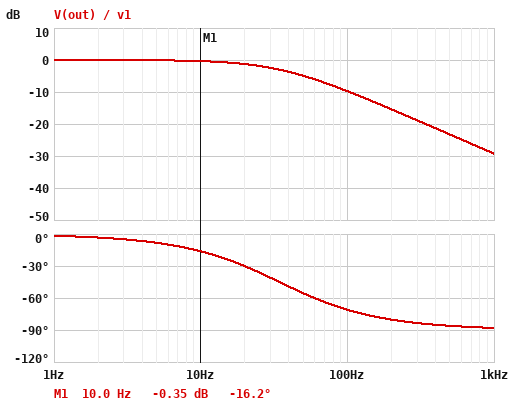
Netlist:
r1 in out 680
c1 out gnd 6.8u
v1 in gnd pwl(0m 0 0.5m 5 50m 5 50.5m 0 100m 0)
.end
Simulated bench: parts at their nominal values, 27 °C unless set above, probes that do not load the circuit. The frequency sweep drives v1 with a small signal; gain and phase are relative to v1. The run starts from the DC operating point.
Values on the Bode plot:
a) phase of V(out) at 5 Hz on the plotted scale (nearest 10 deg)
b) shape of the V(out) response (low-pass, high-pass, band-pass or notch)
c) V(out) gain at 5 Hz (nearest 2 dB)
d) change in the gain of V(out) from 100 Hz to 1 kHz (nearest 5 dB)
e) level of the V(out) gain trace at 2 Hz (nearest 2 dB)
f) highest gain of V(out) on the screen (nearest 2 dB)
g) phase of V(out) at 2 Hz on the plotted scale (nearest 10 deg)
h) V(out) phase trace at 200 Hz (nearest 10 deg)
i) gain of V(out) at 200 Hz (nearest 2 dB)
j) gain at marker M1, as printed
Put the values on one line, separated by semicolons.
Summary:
-10 deg; low-pass; 0 dB; -20 dB; 0 dB; 0 dB; 0 deg; -80 deg; -16 dB; -0.35 dB
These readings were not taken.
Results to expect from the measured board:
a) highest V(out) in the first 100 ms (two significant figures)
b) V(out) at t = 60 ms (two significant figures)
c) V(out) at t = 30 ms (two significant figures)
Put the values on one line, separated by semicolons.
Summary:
5.0 V; 610 mV; 5.0 V
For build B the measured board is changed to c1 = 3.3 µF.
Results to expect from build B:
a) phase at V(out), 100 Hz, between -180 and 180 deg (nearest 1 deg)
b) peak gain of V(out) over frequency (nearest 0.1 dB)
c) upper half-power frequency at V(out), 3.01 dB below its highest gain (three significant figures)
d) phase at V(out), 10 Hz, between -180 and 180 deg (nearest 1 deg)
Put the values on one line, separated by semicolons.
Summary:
-55 deg; 0 dB; 70.9 Hz; -8 deg
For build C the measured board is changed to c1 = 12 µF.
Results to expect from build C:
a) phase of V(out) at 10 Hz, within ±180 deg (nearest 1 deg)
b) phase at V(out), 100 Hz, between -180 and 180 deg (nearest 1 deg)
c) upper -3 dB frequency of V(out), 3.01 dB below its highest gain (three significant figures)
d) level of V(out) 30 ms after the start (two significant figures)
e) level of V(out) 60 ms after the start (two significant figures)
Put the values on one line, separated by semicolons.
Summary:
-27 deg; -79 deg; 19.5 Hz; 4.9 V; 1.5 V
